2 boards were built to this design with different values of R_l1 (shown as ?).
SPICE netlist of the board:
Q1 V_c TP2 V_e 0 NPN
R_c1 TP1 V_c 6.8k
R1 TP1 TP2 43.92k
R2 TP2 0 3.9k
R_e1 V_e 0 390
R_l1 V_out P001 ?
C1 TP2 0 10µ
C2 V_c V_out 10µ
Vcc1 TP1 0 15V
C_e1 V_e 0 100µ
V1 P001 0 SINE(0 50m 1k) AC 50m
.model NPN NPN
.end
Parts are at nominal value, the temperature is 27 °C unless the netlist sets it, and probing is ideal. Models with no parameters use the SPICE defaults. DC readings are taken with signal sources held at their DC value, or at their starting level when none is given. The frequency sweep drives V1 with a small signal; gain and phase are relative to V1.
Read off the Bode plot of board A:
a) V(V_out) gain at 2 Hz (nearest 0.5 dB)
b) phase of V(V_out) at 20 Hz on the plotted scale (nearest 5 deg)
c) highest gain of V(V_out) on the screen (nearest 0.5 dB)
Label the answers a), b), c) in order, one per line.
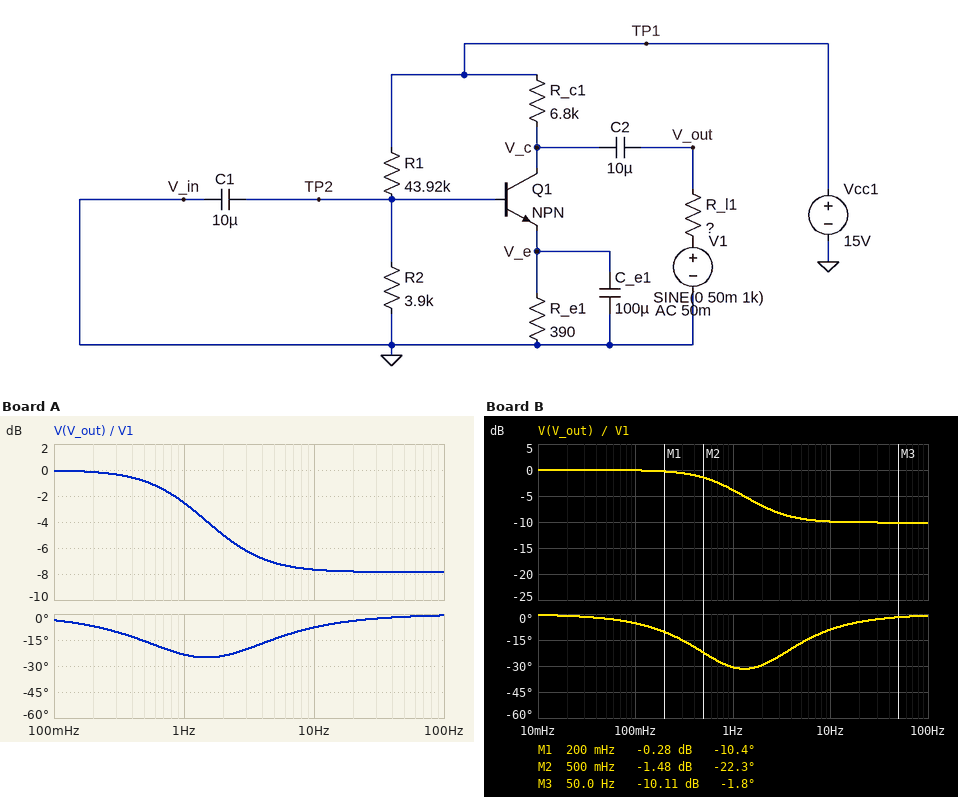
a) -5.0 dB
b) -5 deg
c) 0 dB
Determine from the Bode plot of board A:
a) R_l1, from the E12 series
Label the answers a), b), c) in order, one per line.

a) 10 kΩ
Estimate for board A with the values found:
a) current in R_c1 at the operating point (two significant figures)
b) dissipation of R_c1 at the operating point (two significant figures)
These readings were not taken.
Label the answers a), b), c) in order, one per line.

a) 1.0 mA
b) 7.4 mW
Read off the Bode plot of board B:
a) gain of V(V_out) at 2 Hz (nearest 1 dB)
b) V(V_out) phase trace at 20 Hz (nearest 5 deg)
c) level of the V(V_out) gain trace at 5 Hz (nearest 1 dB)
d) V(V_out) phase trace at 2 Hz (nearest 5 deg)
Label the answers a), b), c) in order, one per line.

a) -7 dB
b) -5 deg
c) -9 dB
d) -30 deg
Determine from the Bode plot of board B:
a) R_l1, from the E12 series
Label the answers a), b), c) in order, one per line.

a) 15 kΩ
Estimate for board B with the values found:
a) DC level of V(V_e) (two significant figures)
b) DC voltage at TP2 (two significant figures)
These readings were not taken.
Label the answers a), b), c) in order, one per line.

a) 410 mV
b) 1.2 V
